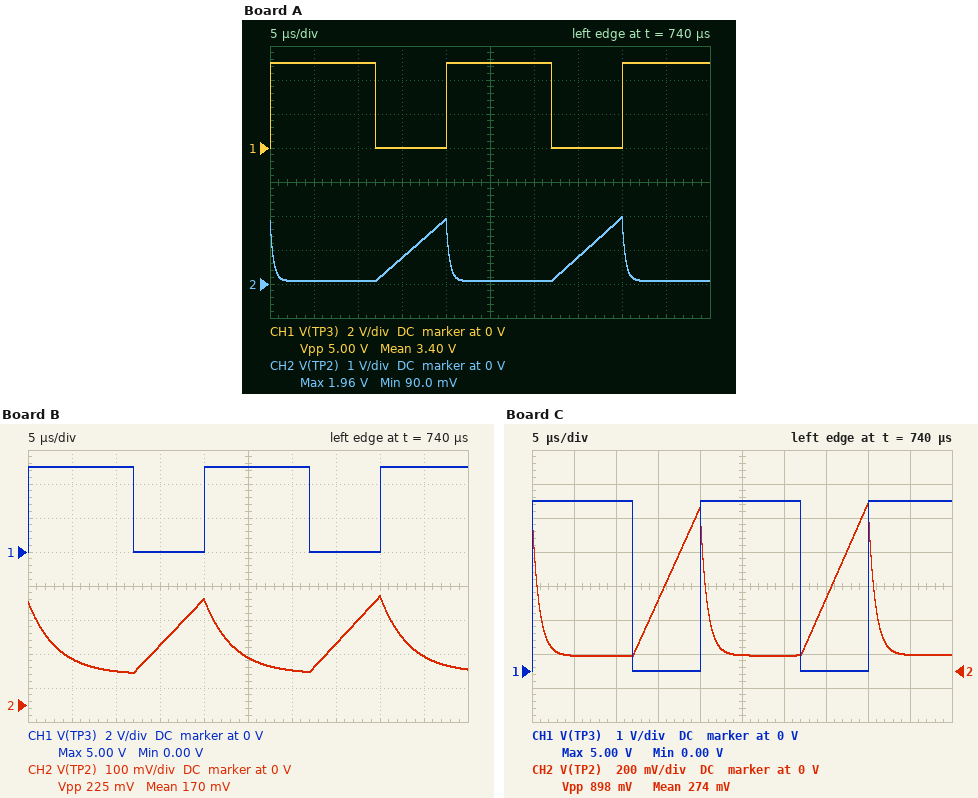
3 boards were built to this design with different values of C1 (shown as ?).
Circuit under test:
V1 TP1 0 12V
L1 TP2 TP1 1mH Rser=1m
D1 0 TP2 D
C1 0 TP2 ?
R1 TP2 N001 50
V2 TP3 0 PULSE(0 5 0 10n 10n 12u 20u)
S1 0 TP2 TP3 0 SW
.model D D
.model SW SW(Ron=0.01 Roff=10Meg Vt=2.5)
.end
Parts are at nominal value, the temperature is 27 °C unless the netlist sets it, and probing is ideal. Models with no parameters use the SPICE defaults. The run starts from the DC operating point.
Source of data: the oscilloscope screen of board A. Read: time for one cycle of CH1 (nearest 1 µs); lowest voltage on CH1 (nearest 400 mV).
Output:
20 µs
0 V
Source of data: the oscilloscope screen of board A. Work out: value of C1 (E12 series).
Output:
39 µF
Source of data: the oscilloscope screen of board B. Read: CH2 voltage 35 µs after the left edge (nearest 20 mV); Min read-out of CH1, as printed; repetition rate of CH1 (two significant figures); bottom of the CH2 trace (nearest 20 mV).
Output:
180 mV
0.00 V
50 kHz
100 mV
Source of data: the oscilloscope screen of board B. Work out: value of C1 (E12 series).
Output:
330 µF
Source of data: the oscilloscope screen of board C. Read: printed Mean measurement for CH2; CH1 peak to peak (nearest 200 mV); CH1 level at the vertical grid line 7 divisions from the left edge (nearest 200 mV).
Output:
274 mV
5.0 V
0 V
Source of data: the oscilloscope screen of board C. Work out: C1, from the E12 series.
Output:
82 µF
